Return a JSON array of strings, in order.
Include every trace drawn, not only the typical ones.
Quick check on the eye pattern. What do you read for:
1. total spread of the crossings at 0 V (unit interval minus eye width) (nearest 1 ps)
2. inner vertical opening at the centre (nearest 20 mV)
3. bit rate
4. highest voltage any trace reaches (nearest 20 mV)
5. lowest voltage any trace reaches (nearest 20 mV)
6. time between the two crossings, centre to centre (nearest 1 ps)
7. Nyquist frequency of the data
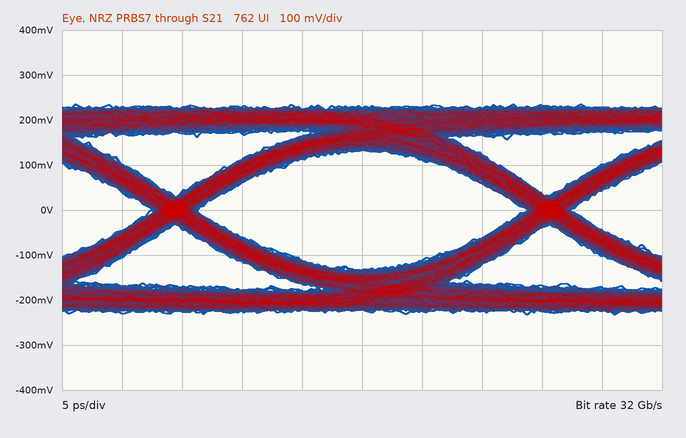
["4 ps", "260 mV", "32 Gb/s", "240 mV", "-240 mV", "31 ps", "16 GHz"]
